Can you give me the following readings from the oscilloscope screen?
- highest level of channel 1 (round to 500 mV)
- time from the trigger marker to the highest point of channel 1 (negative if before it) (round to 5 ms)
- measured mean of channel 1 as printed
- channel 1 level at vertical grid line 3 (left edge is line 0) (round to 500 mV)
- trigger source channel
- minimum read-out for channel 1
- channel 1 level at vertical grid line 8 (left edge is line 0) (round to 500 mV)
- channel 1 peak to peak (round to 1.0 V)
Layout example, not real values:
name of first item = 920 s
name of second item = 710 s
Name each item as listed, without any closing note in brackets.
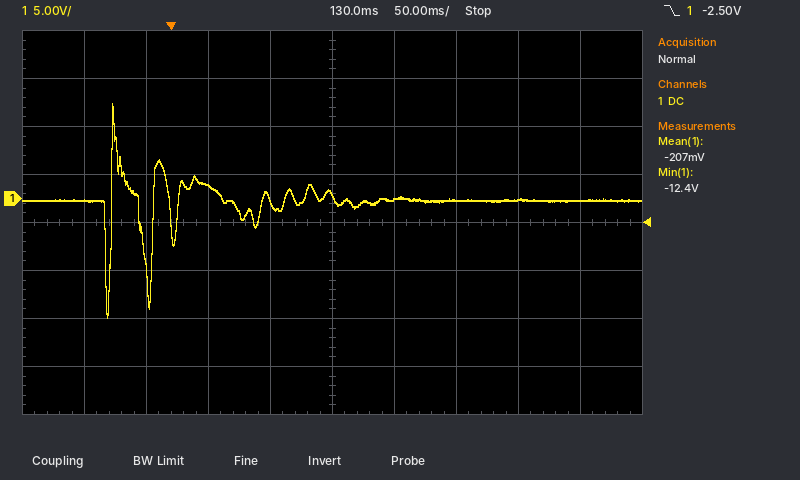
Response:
highest level of channel 1 = 10.0 V
time from the trigger marker to the highest point of channel 1 (negative if before it) = -45 ms
measured mean of channel 1 as printed = -207 mV
channel 1 level at vertical grid line 3 (left edge is line 0) = 1.5 V
trigger source channel = channel 1
minimum read-out for channel 1 = -12.4 V
channel 1 level at vertical grid line 8 (left edge is line 0) = 0.0 V
channel 1 peak to peak = 22.0 V
